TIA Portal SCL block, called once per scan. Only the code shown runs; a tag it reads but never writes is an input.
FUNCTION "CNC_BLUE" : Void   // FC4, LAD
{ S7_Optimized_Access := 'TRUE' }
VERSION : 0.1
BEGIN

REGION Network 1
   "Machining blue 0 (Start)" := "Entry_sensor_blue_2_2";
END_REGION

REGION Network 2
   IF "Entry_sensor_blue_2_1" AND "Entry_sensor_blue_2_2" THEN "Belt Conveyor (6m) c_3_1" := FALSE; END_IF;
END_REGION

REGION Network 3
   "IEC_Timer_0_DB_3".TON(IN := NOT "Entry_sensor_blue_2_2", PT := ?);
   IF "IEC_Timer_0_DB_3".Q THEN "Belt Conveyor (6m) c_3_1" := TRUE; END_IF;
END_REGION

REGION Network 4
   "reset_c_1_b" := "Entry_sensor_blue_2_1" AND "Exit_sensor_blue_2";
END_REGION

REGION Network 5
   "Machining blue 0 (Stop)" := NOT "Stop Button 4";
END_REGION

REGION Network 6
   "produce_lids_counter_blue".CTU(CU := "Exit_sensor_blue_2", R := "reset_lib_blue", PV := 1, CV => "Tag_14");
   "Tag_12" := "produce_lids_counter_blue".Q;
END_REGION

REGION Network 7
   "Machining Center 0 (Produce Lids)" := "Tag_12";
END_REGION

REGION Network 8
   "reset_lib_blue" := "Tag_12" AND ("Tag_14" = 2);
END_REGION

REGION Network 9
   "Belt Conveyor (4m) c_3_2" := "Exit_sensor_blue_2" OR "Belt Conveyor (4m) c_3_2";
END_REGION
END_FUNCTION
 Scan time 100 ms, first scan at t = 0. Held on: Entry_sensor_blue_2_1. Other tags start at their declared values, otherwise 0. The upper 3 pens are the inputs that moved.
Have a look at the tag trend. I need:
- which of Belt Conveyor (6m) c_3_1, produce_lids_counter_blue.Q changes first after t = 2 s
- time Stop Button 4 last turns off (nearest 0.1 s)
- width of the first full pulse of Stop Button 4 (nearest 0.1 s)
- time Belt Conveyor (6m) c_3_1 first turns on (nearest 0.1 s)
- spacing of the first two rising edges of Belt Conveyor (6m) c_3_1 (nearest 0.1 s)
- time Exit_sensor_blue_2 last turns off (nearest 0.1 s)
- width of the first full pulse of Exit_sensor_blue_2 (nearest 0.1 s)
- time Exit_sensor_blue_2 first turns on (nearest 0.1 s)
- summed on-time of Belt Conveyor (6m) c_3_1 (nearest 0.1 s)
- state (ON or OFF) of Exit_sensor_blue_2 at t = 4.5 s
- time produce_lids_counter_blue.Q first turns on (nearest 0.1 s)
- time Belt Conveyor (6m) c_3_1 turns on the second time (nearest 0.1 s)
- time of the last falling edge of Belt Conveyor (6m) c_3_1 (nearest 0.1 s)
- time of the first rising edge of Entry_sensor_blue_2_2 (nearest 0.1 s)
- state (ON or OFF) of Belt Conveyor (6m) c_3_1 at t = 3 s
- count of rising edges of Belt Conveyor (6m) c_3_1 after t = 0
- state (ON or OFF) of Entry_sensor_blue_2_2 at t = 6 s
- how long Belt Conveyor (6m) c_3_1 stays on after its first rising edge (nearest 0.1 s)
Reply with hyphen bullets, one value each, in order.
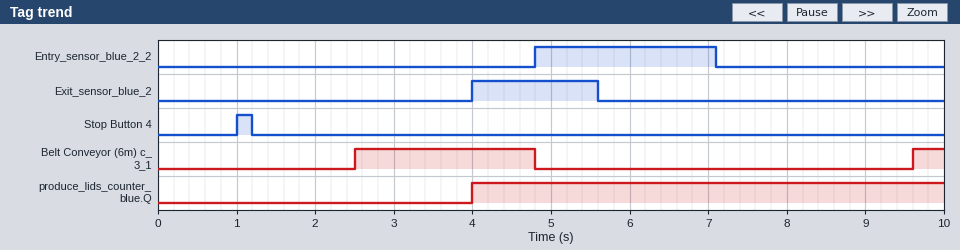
- Belt Conveyor (6m) c_3_1
- 1.2 s
- 0.2 s
- 2.5 s
- 7.1 s
- 5.6 s
- 1.6 s
- 4.0 s
- 2.7 s
- ON
- 4.0 s
- 9.6 s
- 4.8 s
- 4.8 s
- ON
- 2
- ON
- 2.3 s
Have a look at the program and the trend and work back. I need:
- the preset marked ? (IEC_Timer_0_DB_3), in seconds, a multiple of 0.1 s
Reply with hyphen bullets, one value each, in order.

- 2.5 s
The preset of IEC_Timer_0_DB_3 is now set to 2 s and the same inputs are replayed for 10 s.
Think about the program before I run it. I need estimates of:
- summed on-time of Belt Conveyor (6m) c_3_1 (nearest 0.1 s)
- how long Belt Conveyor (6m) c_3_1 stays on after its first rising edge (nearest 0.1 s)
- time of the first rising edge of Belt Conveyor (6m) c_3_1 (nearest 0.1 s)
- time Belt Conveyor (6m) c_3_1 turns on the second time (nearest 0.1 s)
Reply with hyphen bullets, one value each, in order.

- 3.7 s
- 2.8 s
- 2.0 s
- 9.1 s
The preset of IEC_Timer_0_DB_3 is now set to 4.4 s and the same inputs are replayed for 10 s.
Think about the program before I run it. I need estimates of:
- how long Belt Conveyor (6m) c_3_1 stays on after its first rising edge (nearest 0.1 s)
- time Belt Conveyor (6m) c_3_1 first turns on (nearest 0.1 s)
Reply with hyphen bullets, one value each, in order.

- 0.4 s
- 4.4 s
